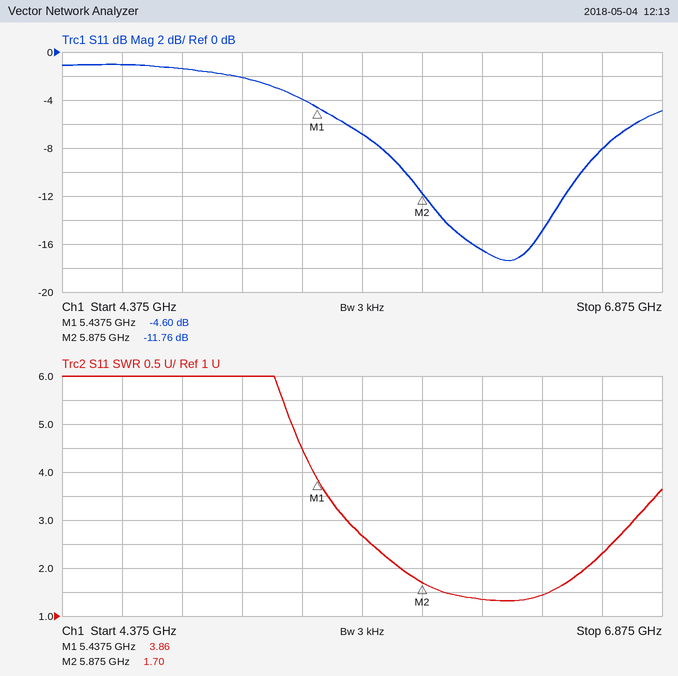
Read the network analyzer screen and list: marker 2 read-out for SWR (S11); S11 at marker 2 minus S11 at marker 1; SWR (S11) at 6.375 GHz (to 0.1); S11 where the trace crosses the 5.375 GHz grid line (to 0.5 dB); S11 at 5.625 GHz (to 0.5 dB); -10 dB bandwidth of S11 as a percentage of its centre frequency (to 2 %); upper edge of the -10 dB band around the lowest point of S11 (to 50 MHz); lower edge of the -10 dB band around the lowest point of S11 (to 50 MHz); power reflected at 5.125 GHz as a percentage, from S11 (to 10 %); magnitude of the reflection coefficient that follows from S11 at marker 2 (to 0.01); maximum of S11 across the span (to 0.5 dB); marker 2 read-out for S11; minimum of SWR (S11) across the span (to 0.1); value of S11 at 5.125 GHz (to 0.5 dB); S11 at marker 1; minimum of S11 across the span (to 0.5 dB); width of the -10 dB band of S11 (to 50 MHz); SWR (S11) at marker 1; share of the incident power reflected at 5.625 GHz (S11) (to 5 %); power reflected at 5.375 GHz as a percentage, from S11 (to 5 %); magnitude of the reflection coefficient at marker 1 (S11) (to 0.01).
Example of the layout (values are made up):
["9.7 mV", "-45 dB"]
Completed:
["1.70", "-7.16 dB", "1.4", "-4.0 dB", "-7.0 dB", "12 %", "6.55 GHz", "5.80 GHz", "60 %", "0.26", "-1.0 dB", "-11.76 dB", "1.3", "-2.0 dB", "-4.60 dB", "-17.5 dB", "750 MHz", "3.86", "20 %", "40 %", "0.59"]
